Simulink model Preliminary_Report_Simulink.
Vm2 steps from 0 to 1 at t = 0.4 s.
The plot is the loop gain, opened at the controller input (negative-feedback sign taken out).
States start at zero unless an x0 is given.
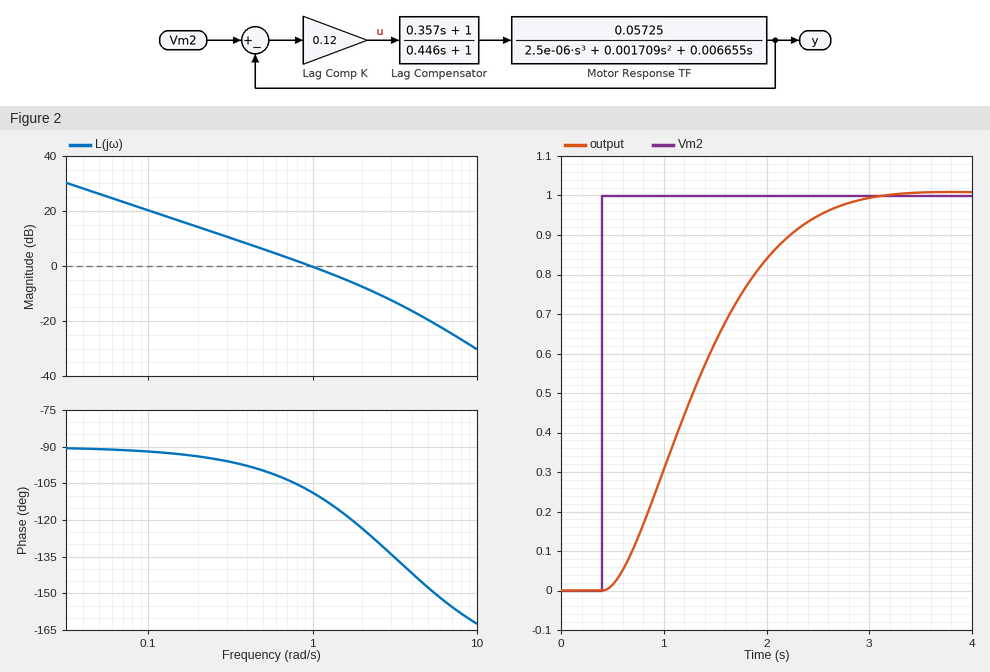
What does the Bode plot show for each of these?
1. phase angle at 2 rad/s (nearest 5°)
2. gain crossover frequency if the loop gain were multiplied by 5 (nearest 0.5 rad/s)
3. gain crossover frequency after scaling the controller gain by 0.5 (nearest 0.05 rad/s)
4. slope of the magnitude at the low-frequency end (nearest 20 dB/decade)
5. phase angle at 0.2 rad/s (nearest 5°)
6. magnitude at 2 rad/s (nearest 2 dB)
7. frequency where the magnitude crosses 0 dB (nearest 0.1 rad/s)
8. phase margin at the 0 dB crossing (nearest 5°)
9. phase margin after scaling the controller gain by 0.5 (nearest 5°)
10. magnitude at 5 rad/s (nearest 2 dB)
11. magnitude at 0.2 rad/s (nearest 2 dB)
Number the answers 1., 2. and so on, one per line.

1. -125°
2. 3.5 rad/s
3. 0.50 rad/s
4. -20 dB/decade
5. -95°
6. -8 dB
7. 1.0 rad/s
8. 70°
9. 80°
10. -20 dB
11. 14 dB
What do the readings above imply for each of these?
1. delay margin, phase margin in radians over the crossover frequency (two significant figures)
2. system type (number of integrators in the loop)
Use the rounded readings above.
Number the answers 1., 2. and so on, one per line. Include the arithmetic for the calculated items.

1. 70 × π / 180 / 1 = 1.2 s
2. 1
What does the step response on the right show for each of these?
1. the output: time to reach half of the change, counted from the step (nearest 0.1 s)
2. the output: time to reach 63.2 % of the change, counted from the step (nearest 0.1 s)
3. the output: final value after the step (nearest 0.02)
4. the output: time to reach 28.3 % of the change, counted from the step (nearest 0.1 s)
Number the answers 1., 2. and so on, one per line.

1. 0.9 s
2. 1.1 s
3. 1.00
4. 0.6 s
